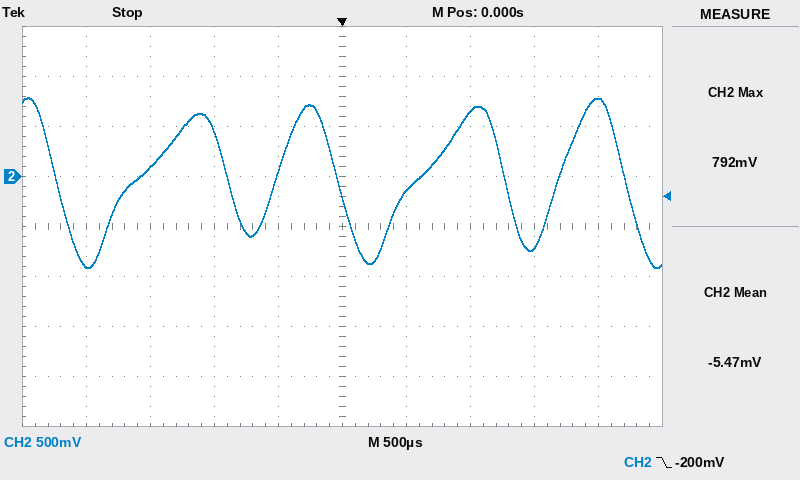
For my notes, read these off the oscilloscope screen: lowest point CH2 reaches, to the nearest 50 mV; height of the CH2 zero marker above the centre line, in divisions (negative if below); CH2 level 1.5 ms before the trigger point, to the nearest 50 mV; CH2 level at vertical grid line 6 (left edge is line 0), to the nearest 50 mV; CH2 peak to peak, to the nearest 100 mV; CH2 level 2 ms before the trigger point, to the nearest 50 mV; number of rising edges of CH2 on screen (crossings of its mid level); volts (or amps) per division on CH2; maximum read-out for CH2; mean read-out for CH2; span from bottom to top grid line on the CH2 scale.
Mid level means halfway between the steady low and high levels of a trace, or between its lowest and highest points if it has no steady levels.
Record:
-900 mV
+1.0 div
100 mV
-150 mV
1.70 V
-900 mV
4
500 mV
792 mV
-5.47 mV
4 V
